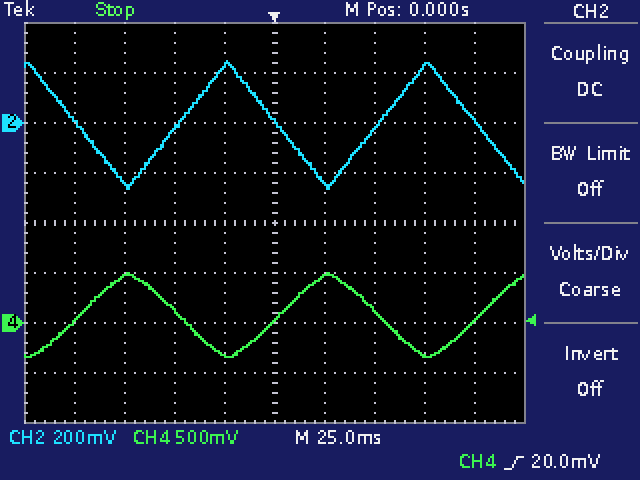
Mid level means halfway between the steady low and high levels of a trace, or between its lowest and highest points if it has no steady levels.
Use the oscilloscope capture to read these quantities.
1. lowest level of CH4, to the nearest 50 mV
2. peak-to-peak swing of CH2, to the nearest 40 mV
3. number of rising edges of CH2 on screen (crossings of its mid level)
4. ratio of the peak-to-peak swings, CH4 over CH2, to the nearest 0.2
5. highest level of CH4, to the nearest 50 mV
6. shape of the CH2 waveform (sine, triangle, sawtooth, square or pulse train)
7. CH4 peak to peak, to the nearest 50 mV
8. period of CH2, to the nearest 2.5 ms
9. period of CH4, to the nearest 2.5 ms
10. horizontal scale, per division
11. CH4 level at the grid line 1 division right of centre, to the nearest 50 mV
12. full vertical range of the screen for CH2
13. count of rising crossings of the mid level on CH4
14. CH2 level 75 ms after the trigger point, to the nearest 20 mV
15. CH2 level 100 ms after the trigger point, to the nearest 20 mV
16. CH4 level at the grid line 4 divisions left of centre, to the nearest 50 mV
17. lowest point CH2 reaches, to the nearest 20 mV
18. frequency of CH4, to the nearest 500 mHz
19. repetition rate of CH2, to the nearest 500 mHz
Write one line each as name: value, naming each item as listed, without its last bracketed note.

lowest level of CH4, to the nearest 50 mV: -350 mV
peak-to-peak swing of CH2, to the nearest 40 mV: 520 mV
number of rising edges of CH2 on screen: 2
ratio of the peak-to-peak swings, CH4 over CH2, to the nearest 0.2: 1.6
highest level of CH4, to the nearest 50 mV: 500 mV
shape of the CH2 waveform: triangle
CH4 peak to peak, to the nearest 50 mV: 850 mV
period of CH2, to the nearest 2.5 ms: 100.0 ms
period of CH4, to the nearest 2.5 ms: 100.0 ms
horizontal scale, per division: 25 ms
CH4 level at the grid line 1 division right of centre, to the nearest 50 mV: 450 mV
full vertical range of the screen for CH2: 1.6 V
count of rising crossings of the mid level on CH4: 3
CH2 level 75 ms after the trigger point, to the nearest 20 mV: 220 mV
CH2 level 100 ms after the trigger point, to the nearest 20 mV: 20 mV
CH4 level at the grid line 4 divisions left of centre, to the nearest 50 mV: 0 mV
lowest point CH2 reaches, to the nearest 20 mV: -260 mV
frequency of CH4, to the nearest 500 mHz: 10.0 Hz
repetition rate of CH2, to the nearest 500 mHz: 10.0 Hz
